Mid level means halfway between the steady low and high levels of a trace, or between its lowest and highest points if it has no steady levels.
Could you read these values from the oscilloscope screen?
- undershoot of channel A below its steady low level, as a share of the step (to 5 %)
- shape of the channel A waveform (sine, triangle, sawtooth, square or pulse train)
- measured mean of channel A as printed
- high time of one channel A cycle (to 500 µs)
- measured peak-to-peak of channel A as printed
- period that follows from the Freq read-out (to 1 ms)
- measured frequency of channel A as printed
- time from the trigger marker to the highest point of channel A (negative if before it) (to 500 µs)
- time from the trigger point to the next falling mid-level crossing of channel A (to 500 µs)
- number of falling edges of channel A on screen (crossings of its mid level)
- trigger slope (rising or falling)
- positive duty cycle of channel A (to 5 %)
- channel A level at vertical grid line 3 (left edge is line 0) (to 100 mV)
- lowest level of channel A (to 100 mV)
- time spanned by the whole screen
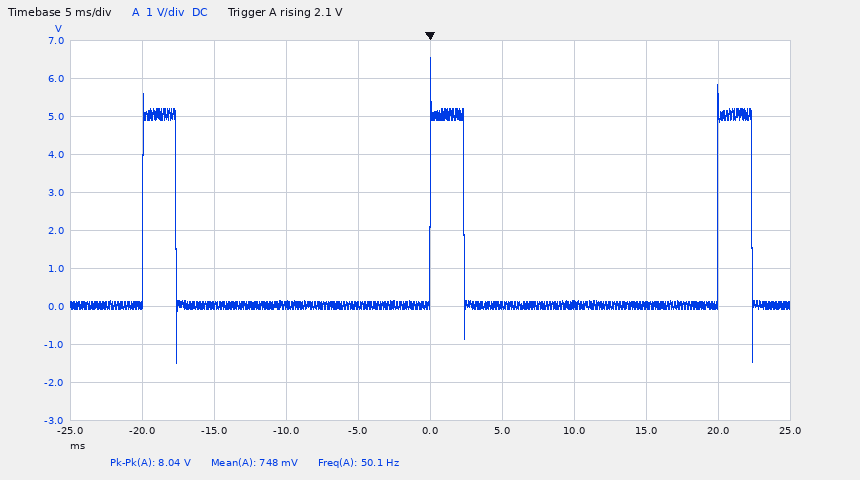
30 %
pulse train
748 mV
2.5 ms
8.04 V
20 ms
50.1 Hz
0.0 ms
2.5 ms
3
rising
10 %
100 mV
-1.5 V
50 ms
